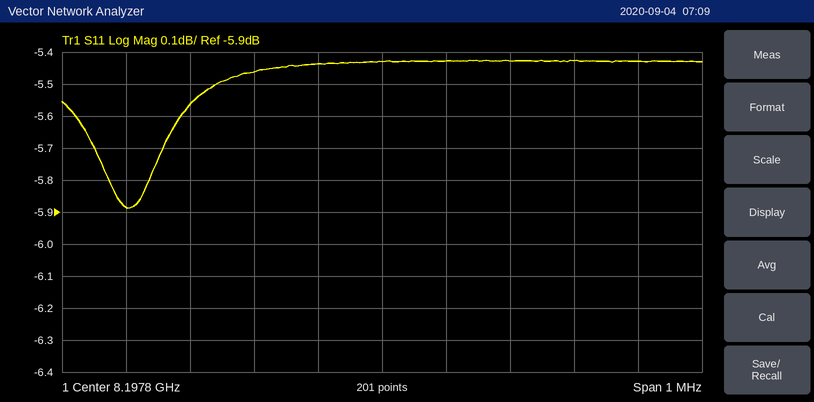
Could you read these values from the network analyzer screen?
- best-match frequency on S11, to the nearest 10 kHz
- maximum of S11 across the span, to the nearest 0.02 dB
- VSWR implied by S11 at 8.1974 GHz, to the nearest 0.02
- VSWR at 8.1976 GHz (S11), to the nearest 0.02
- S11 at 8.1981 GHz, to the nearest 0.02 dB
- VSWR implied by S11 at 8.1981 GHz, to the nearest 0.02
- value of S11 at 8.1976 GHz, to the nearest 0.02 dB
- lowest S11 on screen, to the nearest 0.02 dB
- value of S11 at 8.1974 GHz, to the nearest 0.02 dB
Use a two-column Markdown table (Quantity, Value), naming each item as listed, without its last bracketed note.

| Quantity | Value |
|---|---|
| best-match frequency on S11, to the nearest 10 kHz | 8.19740 GHz |
| maximum of S11 across the span, to the nearest 0.02 dB | -5.42 dB |
| VSWR implied by S11 at 8.1974 GHz, to the nearest 0.02 | 3.06 |
| VSWR at 8.1976 GHz (S11), to the nearest 0.02 | 3.28 |
| S11 at 8.1981 GHz, to the nearest 0.02 dB | -5.42 dB |
| VSWR implied by S11 at 8.1981 GHz, to the nearest 0.02 | 3.30 |
| value of S11 at 8.1976 GHz, to the nearest 0.02 dB | -5.46 dB |
| lowest S11 on screen, to the nearest 0.02 dB | -5.88 dB |
| value of S11 at 8.1974 GHz, to the nearest 0.02 dB | -5.88 dB |
